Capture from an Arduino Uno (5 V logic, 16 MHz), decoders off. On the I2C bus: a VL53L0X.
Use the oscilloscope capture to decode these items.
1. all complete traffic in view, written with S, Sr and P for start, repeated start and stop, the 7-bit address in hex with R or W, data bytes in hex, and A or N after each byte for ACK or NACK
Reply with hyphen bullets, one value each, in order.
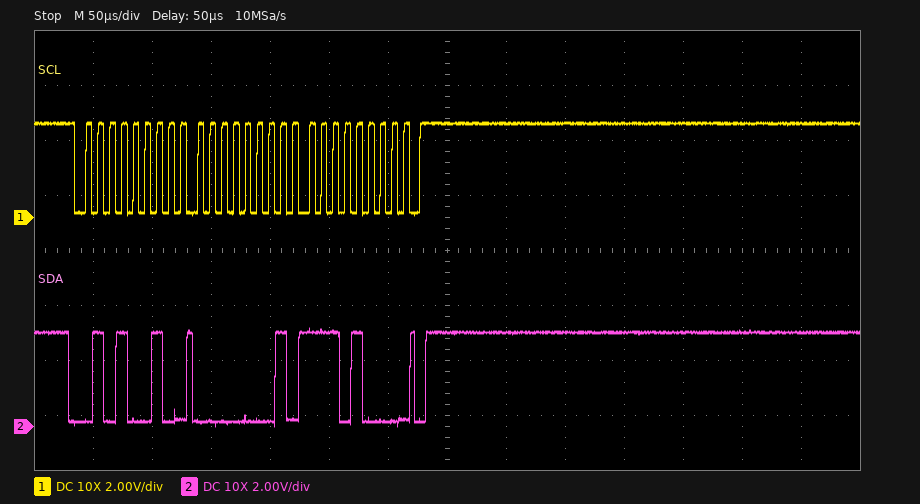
- S 29W A 01 A E8 A P
